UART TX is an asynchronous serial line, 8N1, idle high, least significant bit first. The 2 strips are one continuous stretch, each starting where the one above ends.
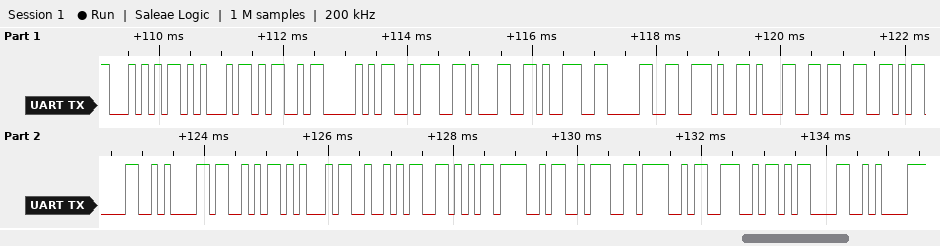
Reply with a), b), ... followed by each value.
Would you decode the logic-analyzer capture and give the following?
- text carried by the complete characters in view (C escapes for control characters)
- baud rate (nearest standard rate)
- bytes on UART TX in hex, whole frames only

a) "TEMP:190.13\r\nSERVO:ON\r\n"
b) 9600 baud
c) 54 45 4D 50 3A 31 39 30 2E 31 33 0D 0A 53 45 52 56 4F 3A 4F 4E 0D 0A
